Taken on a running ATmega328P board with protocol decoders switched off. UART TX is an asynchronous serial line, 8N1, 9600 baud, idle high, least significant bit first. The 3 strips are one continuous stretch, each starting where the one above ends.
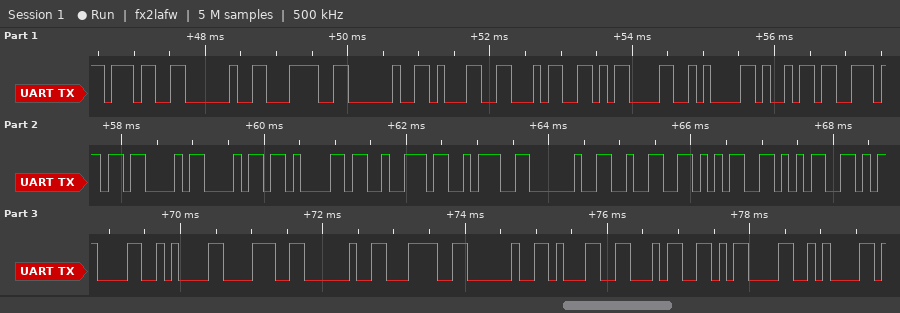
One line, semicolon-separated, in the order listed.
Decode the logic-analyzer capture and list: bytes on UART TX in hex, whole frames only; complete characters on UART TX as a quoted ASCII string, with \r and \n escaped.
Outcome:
37 20 3C 20 31 34 0D 0A 69 6E 43 68 61 72 3A 20 32 35 35 0D 0A 38 20 3C 20 31 34 0D 0A; "7 < 14\r\ninChar: 255\r\n8 < 14\r\n"
